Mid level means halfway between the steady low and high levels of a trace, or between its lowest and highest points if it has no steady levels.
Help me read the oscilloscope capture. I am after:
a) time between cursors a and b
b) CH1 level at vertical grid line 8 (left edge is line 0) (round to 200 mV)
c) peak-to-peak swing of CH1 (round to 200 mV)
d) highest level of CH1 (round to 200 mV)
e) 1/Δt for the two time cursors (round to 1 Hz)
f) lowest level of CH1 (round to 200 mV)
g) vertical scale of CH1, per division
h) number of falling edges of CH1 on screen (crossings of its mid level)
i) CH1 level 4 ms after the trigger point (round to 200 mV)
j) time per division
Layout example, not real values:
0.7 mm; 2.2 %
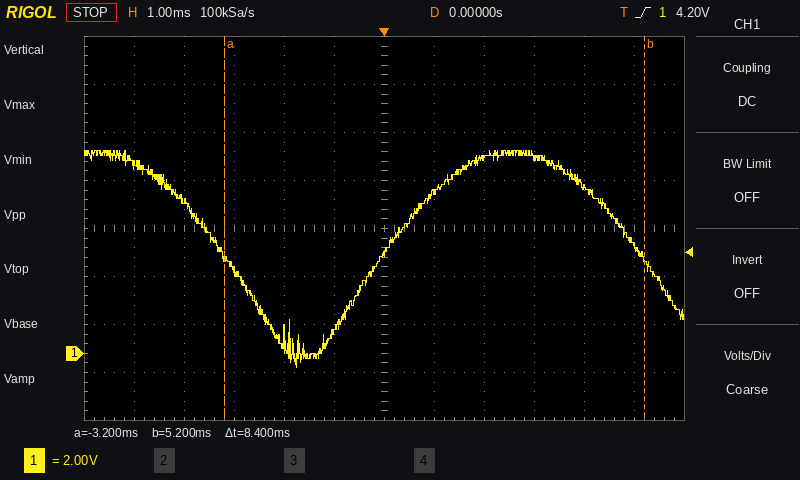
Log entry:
8.4 ms; 8.2 V; 9.0 V; 8.4 V; 119 Hz; -600 mV; 2 V; 2; 7.0 V; 1 ms
